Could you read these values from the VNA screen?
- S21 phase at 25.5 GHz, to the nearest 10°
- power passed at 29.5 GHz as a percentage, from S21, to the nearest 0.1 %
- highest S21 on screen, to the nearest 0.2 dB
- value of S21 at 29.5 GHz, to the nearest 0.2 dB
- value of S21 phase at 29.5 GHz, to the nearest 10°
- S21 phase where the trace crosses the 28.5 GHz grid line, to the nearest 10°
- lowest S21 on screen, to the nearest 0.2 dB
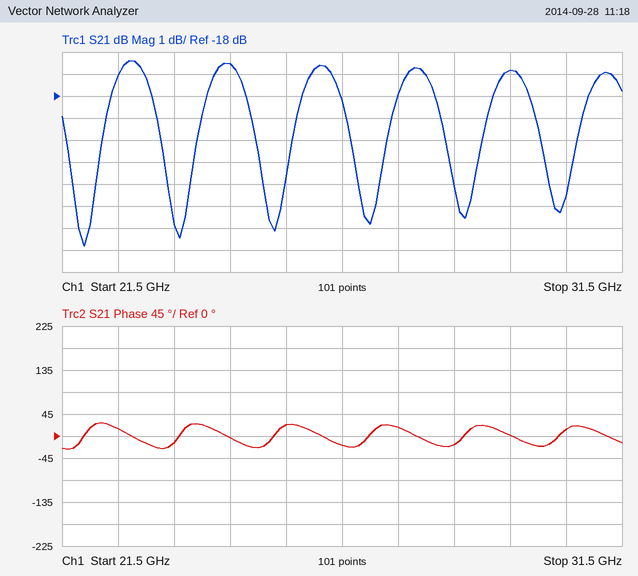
20°
2.1 %
-16.4 dB
-16.8 dB
0°
-20°
-24.8 dB
